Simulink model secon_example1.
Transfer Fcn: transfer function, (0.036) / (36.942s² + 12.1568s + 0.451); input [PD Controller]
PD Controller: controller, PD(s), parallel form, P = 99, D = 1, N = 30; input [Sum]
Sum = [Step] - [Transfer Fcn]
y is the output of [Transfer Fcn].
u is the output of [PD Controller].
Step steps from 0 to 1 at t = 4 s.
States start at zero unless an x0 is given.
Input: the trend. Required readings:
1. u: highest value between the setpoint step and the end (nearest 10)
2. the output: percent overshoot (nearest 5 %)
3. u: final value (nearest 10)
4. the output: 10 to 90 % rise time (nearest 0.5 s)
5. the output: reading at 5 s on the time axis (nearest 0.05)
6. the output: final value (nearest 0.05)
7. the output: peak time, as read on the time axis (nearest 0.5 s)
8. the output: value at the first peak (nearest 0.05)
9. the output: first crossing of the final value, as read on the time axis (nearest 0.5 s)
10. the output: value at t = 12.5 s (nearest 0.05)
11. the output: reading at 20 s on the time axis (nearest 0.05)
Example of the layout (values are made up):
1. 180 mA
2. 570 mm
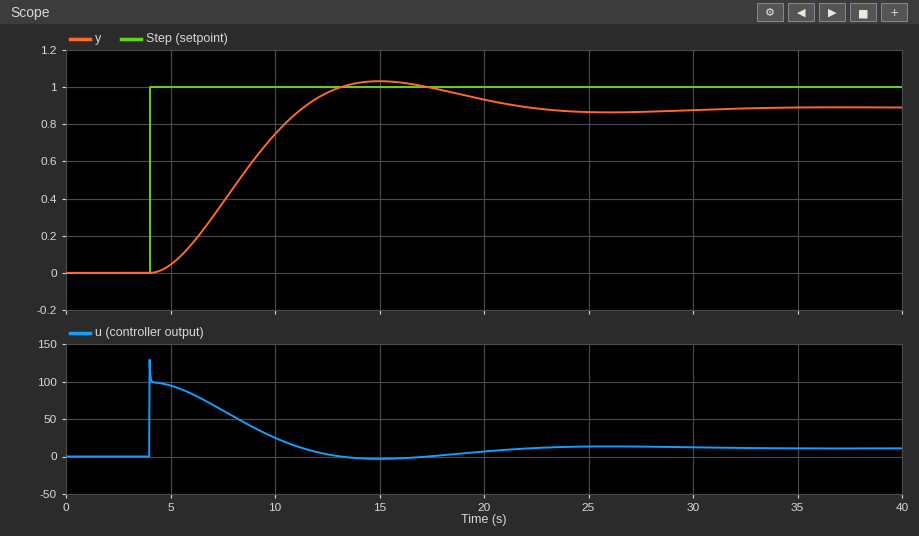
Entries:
1. 130
2. 15 %
3. 10
4. 5.0 s
5. 0.05
6. 0.90
7. 15.0 s
8. 1.05
9. 11.5 s
10. 0.95
11. 0.95
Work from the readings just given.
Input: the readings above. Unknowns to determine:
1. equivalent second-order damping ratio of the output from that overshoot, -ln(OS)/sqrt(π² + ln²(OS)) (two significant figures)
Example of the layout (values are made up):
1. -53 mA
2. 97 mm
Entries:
1. 0.52
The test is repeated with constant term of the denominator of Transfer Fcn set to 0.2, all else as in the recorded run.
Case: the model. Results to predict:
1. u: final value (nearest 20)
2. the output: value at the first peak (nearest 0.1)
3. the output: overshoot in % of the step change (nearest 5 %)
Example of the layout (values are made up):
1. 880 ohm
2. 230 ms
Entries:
1. 0
2. 1.1
3. 15 %
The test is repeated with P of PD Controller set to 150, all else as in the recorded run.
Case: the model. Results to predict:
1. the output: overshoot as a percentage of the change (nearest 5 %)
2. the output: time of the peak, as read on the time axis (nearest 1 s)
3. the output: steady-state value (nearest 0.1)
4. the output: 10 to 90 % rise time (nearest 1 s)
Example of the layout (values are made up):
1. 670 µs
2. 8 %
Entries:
1. 25 %
2. 13 s
3. 0.9
4. 4 s
